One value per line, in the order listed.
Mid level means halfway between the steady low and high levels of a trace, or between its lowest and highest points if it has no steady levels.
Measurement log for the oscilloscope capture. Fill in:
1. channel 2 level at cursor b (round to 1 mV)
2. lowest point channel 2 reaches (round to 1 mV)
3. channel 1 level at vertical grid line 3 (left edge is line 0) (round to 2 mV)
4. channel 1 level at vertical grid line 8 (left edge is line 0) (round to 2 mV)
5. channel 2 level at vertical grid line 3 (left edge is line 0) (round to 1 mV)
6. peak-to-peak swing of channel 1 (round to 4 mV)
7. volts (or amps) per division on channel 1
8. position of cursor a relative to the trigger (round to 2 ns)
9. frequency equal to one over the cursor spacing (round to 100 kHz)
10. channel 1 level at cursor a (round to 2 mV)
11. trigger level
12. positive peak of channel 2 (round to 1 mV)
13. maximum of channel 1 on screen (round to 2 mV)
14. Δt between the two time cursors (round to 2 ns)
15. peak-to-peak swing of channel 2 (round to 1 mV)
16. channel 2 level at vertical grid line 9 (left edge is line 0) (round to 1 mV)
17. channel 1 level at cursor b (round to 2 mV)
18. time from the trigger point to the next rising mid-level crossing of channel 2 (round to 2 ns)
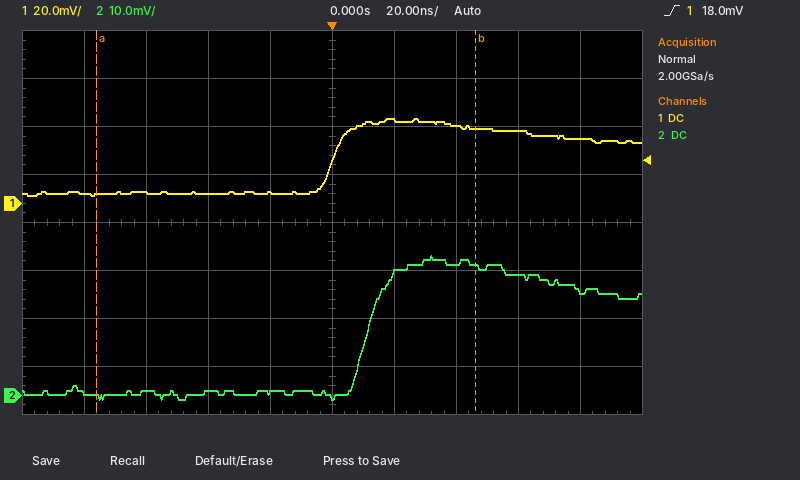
27 mV
-1 mV
4 mV
30 mV
1 mV
32 mV
20 mV
-76 ns
8.2 MHz
4 mV
18.0 mV
29 mV
36 mV
122 ns
30 mV
22 mV
32 mV
12 ns
